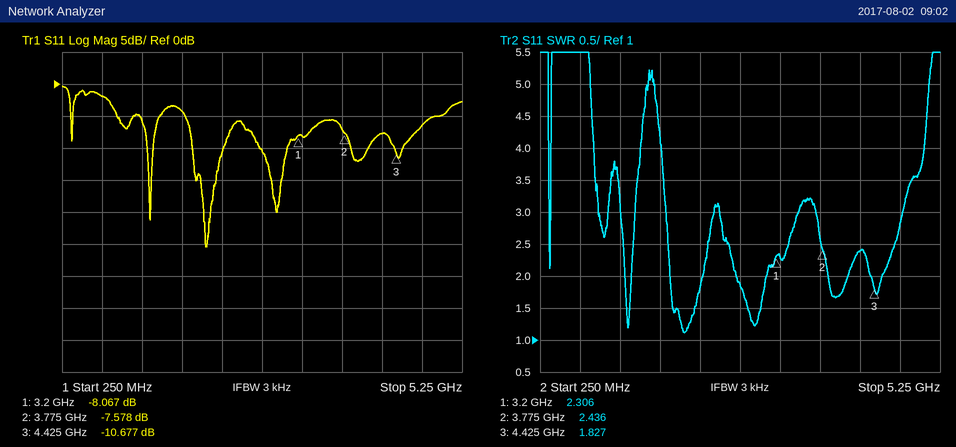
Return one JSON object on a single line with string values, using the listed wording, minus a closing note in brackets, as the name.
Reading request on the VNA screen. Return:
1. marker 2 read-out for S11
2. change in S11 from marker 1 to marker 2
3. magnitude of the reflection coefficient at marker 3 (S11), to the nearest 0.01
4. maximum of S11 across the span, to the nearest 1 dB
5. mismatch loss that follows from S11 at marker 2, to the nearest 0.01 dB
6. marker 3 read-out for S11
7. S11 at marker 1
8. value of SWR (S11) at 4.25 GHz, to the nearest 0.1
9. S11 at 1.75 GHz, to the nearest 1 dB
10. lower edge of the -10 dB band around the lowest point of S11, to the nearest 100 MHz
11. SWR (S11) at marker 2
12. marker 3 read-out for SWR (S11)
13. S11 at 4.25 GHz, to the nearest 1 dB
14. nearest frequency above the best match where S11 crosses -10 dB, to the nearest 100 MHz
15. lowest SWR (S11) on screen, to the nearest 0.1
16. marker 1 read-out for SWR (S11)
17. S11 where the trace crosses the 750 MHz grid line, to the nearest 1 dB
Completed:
{"marker 2 read-out for S11": "-7.578 dB", "change in S11 from marker 1 to marker 2": "0.489 dB", "magnitude of the reflection coefficient at marker 3 (S11), to the nearest 0.01": "0.29", "maximum of S11 across the span, to the nearest 1 dB": "0 dB", "mismatch loss that follows from S11 at marker 2, to the nearest 0.01 dB": "0.83 dB", "marker 3 read-out for S11": "-10.677 dB", "S11 at marker 1": "-8.067 dB", "value of SWR (S11) at 4.25 GHz, to the nearest 0.1": "2.4", "S11 at 1.75 GHz, to the nearest 1 dB": "-4 dB", "lower edge of the -10 dB band around the lowest point of S11, to the nearest 100 MHz": "1.9 GHz", "SWR (S11) at marker 2": "2.436", "marker 3 read-out for SWR": "1.827", "S11 at 4.25 GHz, to the nearest 1 dB": "-8 dB", "nearest frequency above the best match where S11 crosses -10 dB, to the nearest 100 MHz": "2.3 GHz", "lowest SWR (S11) on screen, to the nearest 0.1": "1.1", "marker 1 read-out for SWR": "2.306", "S11 where the trace crosses the 750 MHz grid line, to the nearest 1 dB": "-2 dB"}
